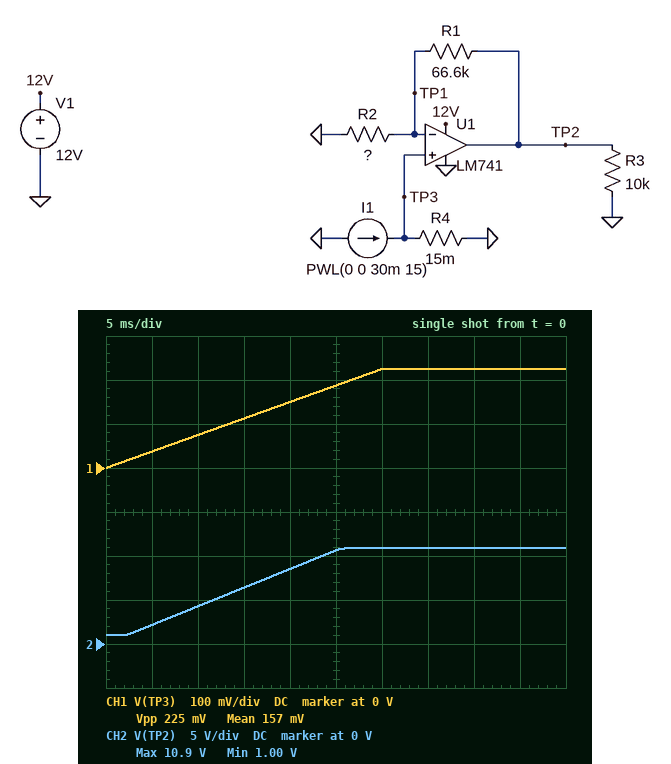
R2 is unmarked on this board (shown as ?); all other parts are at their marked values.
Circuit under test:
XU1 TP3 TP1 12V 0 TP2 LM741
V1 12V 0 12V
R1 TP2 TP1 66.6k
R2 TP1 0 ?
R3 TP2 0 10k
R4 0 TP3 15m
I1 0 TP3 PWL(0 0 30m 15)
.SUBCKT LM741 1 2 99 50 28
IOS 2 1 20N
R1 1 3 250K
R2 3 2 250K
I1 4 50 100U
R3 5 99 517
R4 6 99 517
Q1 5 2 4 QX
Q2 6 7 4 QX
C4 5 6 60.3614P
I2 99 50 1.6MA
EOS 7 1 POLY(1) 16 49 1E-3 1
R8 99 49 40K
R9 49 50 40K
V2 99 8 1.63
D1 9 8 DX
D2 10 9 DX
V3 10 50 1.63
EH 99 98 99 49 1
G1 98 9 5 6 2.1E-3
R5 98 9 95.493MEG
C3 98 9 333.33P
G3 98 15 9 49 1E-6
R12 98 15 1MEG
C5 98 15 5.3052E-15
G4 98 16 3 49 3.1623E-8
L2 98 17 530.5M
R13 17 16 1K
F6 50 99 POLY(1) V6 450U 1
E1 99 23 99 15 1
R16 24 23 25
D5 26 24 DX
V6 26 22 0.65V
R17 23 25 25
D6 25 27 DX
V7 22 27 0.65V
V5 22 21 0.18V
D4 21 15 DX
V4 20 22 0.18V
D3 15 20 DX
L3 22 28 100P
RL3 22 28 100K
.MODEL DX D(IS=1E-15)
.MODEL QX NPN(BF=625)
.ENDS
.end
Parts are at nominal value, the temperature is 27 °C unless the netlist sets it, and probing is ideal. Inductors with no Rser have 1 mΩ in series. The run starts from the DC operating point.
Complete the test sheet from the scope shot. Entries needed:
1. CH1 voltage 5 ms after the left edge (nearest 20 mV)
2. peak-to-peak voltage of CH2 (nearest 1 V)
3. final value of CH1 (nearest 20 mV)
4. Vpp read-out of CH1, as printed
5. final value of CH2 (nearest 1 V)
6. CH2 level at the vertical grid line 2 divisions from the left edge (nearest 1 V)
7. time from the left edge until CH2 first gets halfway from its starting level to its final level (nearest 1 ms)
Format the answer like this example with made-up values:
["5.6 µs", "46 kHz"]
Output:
["40 mV", "10 V", "220 mV", "225 mV", "11 V", "4 V", "14 ms"]
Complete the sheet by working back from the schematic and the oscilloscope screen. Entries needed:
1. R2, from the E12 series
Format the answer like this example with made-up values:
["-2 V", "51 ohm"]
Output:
["1.2 kΩ"]
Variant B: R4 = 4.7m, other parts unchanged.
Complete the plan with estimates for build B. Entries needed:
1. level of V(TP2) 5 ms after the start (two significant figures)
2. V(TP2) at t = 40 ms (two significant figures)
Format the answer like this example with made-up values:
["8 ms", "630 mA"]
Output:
["1.0 V", "4.0 V"]
